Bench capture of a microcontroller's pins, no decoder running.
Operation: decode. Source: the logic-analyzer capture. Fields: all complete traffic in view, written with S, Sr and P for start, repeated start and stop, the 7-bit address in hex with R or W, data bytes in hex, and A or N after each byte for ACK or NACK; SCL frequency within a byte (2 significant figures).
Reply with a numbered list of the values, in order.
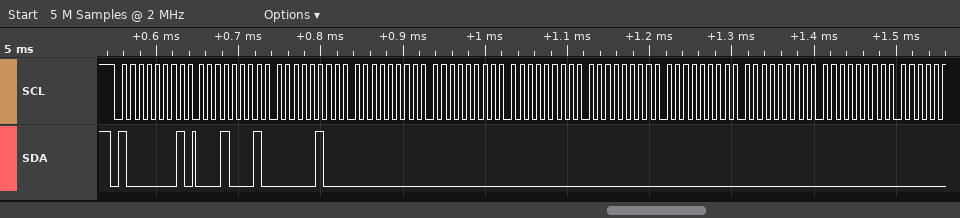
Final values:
1. S 40R A 11 A 04 A 00 A 00 A 00 A 00 A 00 A 00 A 00 A
2. 100 kHz
